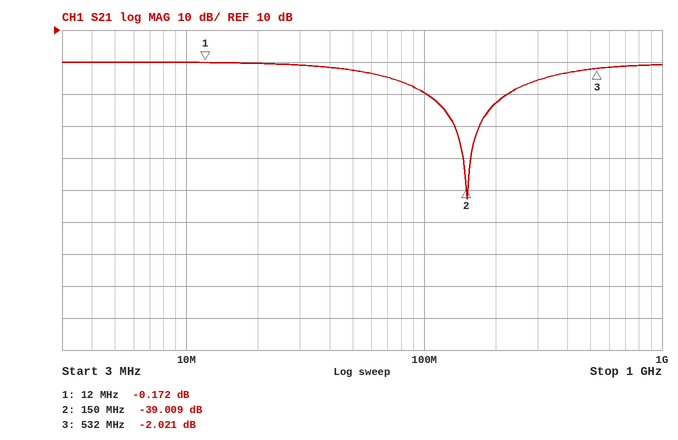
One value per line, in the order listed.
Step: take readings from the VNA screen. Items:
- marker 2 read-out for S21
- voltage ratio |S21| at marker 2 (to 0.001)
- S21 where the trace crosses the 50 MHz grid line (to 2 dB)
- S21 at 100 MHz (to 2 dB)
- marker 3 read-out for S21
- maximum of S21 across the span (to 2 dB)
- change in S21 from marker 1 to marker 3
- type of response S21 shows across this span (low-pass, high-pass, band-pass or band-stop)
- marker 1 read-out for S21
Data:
-39.009 dB
0.011
-2 dB
-10 dB
-2.021 dB
0 dB
-1.849 dB
band-stop
-0.172 dB
